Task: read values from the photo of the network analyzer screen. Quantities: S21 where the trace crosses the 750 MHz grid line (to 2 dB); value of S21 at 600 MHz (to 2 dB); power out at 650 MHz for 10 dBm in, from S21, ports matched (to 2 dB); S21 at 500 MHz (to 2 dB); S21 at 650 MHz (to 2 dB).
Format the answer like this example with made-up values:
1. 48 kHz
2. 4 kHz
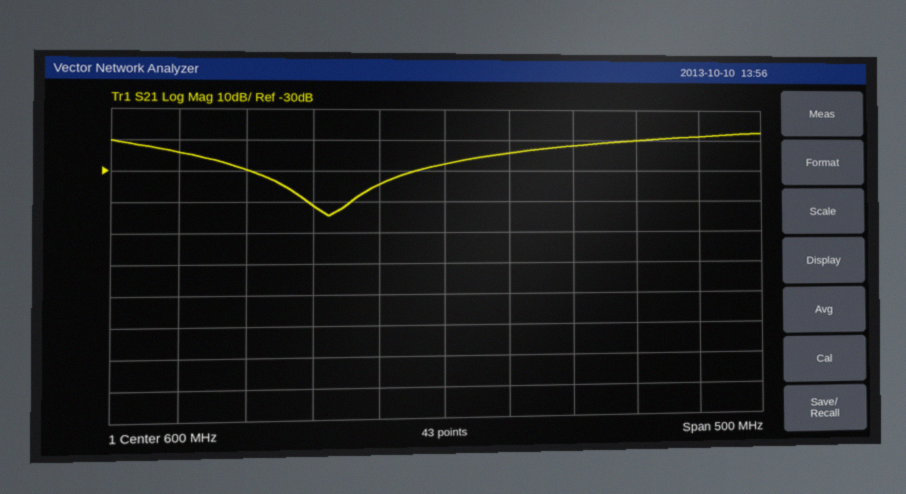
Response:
1. -20 dB
2. -28 dB
3. -14 dBm
4. -42 dB
5. -24 dB
